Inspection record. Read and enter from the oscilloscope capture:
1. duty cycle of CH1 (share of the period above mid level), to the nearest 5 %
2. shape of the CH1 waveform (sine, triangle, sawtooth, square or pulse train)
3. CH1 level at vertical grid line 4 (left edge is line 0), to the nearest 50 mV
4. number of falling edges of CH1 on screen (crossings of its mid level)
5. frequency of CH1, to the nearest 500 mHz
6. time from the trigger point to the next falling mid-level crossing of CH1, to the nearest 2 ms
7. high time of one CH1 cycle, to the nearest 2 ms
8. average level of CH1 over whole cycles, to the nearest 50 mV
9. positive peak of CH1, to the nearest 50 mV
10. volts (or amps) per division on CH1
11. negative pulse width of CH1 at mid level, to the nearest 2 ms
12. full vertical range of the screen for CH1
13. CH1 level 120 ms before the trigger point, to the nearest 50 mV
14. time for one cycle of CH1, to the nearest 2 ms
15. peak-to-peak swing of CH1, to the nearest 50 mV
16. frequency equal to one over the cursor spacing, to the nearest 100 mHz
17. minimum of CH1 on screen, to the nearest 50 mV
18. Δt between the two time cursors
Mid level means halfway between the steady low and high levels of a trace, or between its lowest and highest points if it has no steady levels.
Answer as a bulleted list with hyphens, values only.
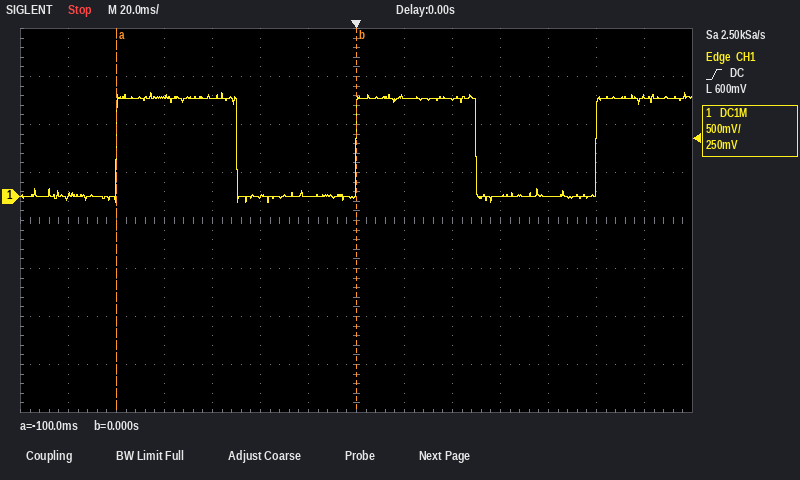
- 50 %
- square
- 1.00 V
- 2
- 10.0 Hz
- 50 ms
- 50 ms
- 500 mV
- 1.10 V
- 500 mV
- 50 ms
- 4 V
- 0 mV
- 100 ms
- 1.15 V
- 10.0 Hz
- -50 mV
- 100 ms
